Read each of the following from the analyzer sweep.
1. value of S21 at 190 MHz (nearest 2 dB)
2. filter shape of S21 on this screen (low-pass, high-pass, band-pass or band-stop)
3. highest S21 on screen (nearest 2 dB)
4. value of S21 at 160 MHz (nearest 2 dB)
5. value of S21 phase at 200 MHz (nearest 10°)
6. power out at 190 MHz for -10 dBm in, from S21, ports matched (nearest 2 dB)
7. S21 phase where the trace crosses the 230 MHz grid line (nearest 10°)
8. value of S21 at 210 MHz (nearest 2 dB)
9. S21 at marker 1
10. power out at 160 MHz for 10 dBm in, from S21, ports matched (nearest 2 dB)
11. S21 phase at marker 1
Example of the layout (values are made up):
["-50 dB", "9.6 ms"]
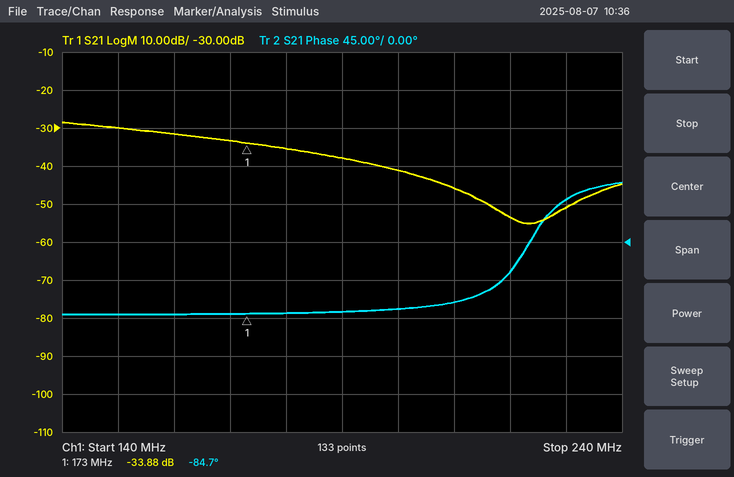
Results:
["-38 dB", "low-pass", "-28 dB", "-32 dB", "-80°", "-48 dBm", "50°", "-46 dB", "-33.88 dB", "-22 dBm", "-84.7°"]
